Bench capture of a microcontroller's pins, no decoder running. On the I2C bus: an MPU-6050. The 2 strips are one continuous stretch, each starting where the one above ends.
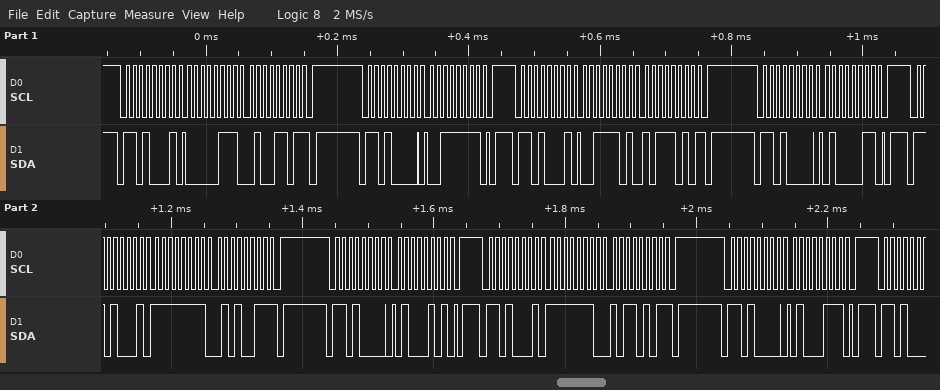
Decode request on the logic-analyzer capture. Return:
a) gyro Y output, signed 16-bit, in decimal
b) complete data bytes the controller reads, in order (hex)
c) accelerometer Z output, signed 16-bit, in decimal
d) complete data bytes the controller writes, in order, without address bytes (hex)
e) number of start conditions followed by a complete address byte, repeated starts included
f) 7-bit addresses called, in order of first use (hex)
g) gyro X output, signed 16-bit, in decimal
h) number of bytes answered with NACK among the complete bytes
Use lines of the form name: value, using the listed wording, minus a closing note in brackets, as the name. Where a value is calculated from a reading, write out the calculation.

gyro Y output, signed 16-bit, in decimal: 0xFEB5 = -331
complete data bytes the controller reads, in order: 07 4D 3D BA FF 53 FE B5
accelerometer Z output, signed 16-bit, in decimal: 0x3DBA = 15802
complete data bytes the controller writes, in order, without address bytes: 3F 43 45 47
number of start conditions followed by a complete address byte, repeated starts included: 8
7-bit addresses called, in order of first use: 0x68
gyro X output, signed 16-bit, in decimal: 0xFF53 = -173
number of bytes answered with NACK among the complete bytes: 4
